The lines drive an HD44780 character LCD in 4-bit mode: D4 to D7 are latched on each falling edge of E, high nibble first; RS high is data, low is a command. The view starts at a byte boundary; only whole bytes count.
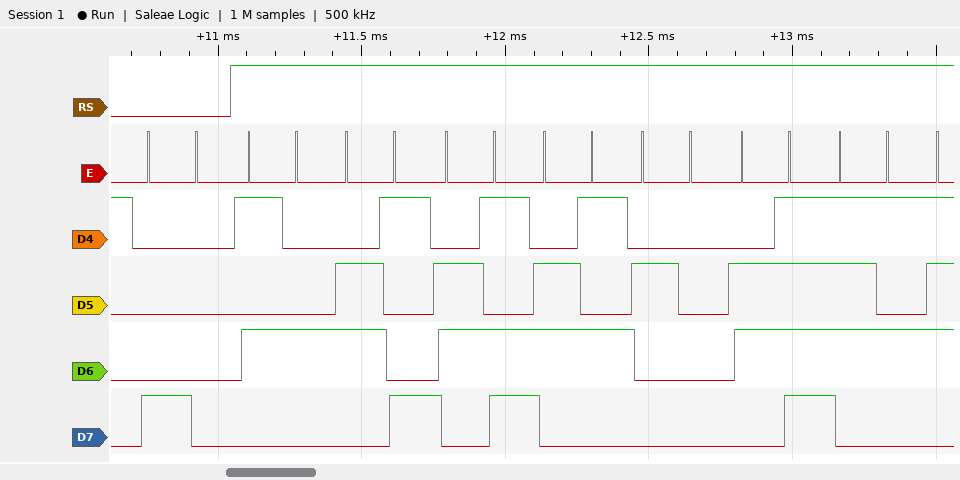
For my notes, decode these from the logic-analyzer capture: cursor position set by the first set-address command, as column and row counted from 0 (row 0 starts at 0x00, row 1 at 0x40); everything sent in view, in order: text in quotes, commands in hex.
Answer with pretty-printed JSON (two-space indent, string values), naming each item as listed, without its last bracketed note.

{
  "cursor position set by the first set-address command, as column and row counted from 0": "column 0, row 0",
  "everything sent in view, in order: text in quotes, commands in hex": "0x80 \"Time ou\""
}
